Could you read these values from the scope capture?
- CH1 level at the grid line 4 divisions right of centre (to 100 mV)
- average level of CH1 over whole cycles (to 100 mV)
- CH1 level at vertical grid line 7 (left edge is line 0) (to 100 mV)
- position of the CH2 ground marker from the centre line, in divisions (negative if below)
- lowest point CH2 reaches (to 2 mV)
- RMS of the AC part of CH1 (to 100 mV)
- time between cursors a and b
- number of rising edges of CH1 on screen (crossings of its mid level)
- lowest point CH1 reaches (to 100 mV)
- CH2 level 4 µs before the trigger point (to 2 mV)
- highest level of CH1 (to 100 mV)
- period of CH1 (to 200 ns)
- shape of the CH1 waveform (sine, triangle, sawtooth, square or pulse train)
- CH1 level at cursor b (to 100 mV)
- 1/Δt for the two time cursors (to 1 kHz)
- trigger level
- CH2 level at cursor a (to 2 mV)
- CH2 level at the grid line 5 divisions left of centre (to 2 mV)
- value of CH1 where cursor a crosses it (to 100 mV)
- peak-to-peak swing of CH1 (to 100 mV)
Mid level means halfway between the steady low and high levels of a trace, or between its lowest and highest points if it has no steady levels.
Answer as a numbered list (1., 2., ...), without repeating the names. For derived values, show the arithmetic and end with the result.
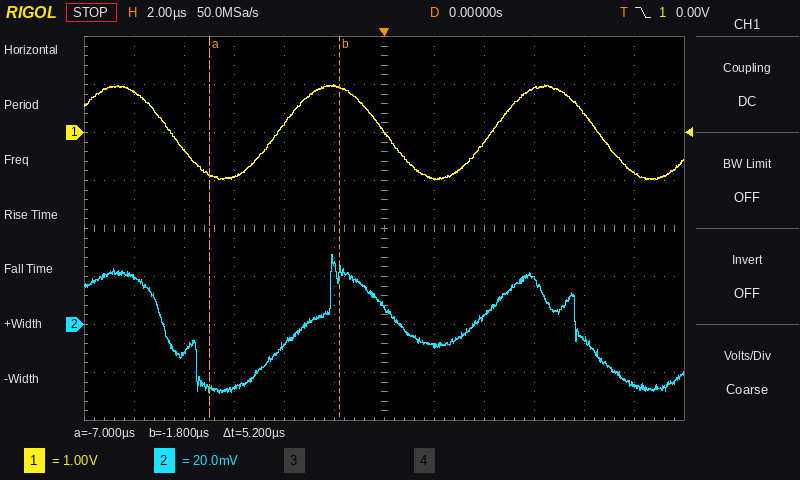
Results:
1. 400 mV
2. (1.0 V + (-1.0 V)) / 2 ≈ 0.0 V
3. -1.0 V
4. -2.0 div
5. -28 mV
6. 2.0 V / (2√2) ≈ 707 mV, so 700 mV to the nearest 100 mV
7. 5.2 µs
8. 2
9. -1.0 V
10. -8 mV
11. 1.0 V
12. 8.6 µs
13. sine
14. 900 mV
15. 1 / 5.2 µs ≈ 192 kHz
16. 0.00 V
17. -26 mV
18. 20 mV
19. -900 mV
20. 1.0 V − (-1.0 V) = 2.0 V
